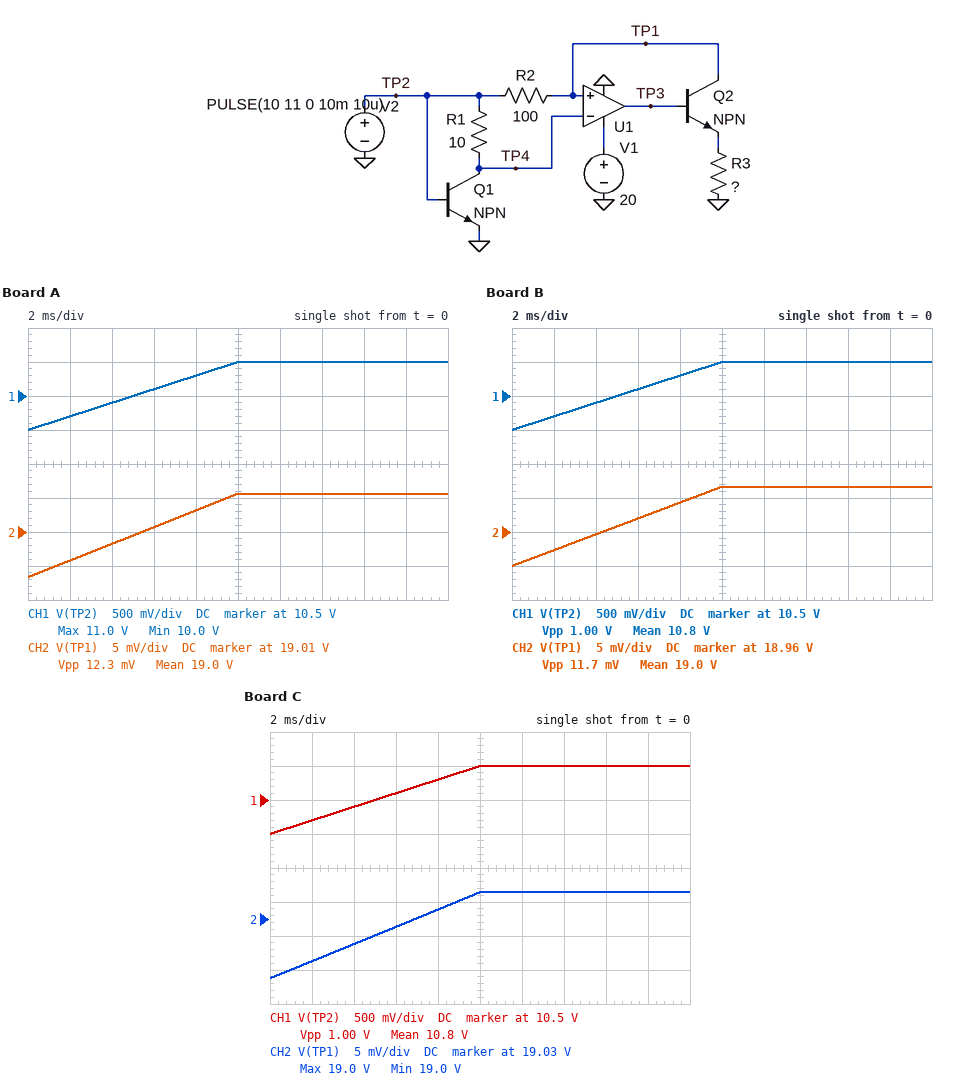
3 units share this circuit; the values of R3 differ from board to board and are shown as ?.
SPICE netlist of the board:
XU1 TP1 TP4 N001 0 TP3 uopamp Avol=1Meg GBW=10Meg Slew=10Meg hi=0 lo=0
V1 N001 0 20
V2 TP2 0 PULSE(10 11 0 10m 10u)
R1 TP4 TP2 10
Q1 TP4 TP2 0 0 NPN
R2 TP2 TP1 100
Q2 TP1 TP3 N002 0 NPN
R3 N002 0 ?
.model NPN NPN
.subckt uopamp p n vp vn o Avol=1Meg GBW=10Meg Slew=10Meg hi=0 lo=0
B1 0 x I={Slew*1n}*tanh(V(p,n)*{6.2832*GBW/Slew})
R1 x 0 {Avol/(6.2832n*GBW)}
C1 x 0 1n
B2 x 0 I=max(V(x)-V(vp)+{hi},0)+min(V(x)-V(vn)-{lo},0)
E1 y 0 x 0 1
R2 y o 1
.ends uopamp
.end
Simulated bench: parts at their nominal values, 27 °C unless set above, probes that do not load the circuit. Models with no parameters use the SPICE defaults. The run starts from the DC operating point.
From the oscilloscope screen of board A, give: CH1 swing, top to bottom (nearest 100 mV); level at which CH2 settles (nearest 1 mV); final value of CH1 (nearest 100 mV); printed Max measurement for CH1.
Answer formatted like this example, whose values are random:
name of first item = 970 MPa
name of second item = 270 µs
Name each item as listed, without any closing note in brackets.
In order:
CH1 swing, top to bottom = 1.0 V
level at which CH2 settles = 19.016 V
final value of CH1 = 11.0 V
printed Max measurement for CH1 = 11.0 V
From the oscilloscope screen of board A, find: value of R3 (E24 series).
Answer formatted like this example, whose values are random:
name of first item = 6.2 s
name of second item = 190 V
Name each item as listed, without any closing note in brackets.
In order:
value of R3 = 910 Ω
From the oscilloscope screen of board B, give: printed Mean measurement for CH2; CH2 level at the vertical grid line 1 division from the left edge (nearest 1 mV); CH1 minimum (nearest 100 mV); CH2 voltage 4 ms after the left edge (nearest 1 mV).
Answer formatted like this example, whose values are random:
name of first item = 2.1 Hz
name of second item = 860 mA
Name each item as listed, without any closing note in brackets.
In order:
printed Mean measurement for CH2 = 19.0 V
CH2 level at the vertical grid line 1 division from the left edge = 18.962 V
CH1 minimum = 10.0 V
CH2 voltage 4 ms after the left edge = 18.965 V
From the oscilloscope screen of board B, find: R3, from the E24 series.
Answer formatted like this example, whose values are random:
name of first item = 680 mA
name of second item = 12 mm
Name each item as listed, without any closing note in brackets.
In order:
R3, from the E24 series = 330 Ω
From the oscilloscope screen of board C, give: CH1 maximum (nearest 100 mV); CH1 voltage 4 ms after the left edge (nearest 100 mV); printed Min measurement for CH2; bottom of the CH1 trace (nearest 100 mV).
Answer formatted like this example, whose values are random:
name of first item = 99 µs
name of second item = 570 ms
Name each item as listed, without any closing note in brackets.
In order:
CH1 maximum = 11.0 V
CH1 voltage 4 ms after the left edge = 10.4 V
printed Min measurement for CH2 = 19.0 V
bottom of the CH1 trace = 10.0 V
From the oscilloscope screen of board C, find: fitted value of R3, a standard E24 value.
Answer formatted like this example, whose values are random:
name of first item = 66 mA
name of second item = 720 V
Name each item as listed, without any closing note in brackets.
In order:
fitted value of R3, a standard E24 value = 3 kΩ
